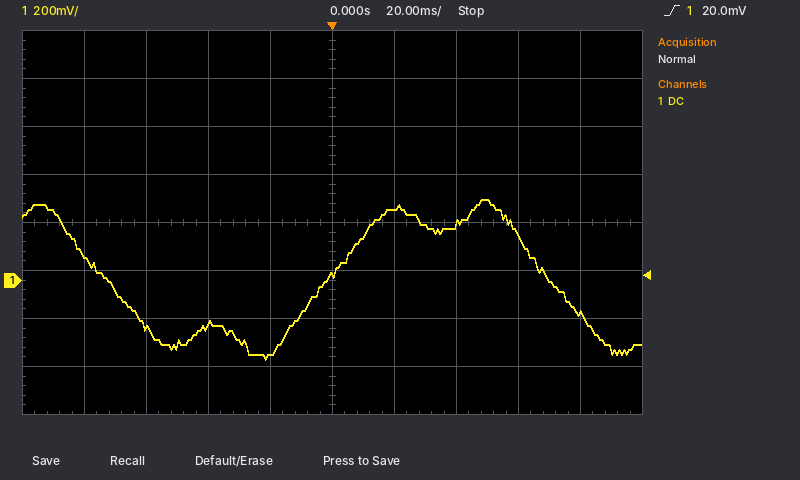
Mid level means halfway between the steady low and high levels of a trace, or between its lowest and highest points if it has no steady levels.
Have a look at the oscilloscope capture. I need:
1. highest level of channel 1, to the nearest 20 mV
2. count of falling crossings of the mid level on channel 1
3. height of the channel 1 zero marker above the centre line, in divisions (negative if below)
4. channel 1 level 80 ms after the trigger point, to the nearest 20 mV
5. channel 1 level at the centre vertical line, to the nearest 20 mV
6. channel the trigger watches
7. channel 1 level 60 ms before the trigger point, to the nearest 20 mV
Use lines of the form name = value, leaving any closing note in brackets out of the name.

highest level of channel 1, to the nearest 20 mV = 340 mV
count of falling crossings of the mid level on channel 1 = 2
height of the channel 1 zero marker above the centre line, in divisions = -1.2 div
channel 1 level 80 ms after the trigger point, to the nearest 20 mV = -140 mV
channel 1 level at the centre vertical line, to the nearest 20 mV = 20 mV
channel the trigger watches = channel 1
channel 1 level 60 ms before the trigger point, to the nearest 20 mV = -200 mV
